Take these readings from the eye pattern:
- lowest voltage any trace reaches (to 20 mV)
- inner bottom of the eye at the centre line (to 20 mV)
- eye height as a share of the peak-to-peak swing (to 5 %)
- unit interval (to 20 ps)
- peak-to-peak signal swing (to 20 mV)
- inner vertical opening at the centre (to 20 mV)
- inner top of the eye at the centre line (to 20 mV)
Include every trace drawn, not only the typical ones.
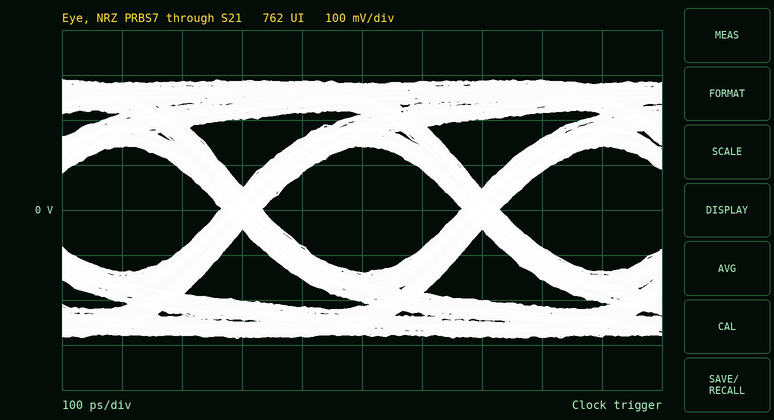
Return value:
-280 mV
-140 mV
50 %
400 ps
580 mV
280 mV
140 mV
